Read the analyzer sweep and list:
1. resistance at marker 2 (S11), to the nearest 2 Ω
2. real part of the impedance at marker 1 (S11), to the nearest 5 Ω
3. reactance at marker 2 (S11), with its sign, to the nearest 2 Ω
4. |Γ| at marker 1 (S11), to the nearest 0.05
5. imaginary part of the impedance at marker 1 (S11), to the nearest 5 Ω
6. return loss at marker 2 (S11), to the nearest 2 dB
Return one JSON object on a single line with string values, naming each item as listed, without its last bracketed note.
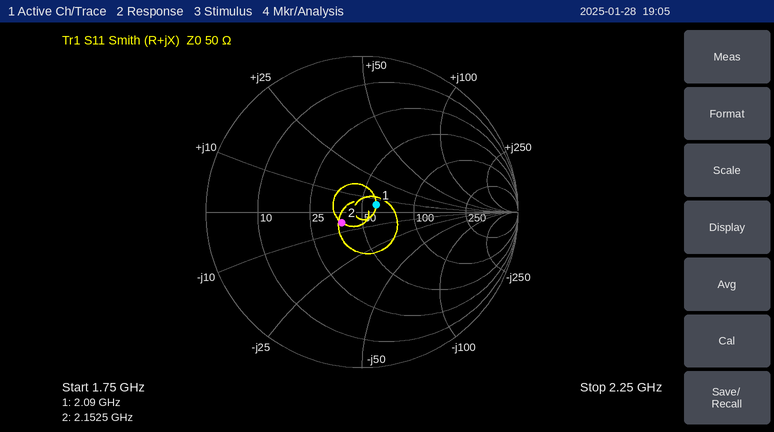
{"resistance at marker 2 (S11), to the nearest 2 Ω": "38 Ω", "real part of the impedance at marker 1 (S11), to the nearest 5 Ω": "60 Ω", "reactance at marker 2 (S11), with its sign, to the nearest 2 Ω": "-6 Ω", "|Γ| at marker 1 (S11), to the nearest 0.05": "0.10", "imaginary part of the impedance at marker 1 (S11), to the nearest 5 Ω": "+5 Ω", "return loss at marker 2 (S11), to the nearest 2 dB": "16 dB"}
